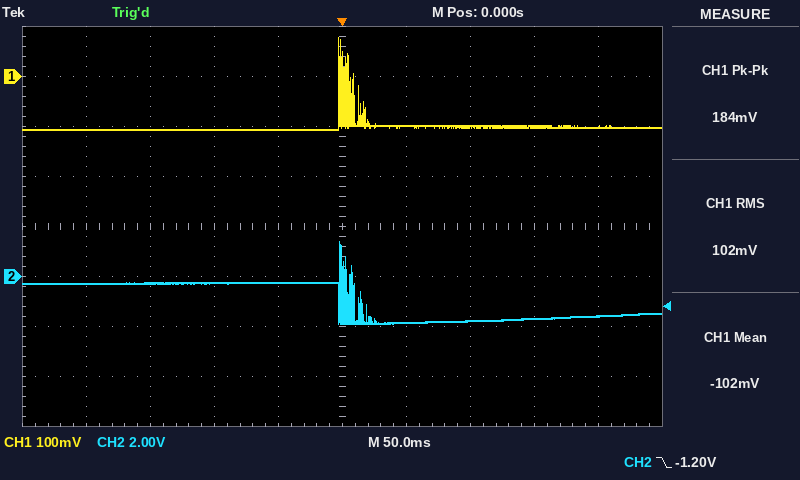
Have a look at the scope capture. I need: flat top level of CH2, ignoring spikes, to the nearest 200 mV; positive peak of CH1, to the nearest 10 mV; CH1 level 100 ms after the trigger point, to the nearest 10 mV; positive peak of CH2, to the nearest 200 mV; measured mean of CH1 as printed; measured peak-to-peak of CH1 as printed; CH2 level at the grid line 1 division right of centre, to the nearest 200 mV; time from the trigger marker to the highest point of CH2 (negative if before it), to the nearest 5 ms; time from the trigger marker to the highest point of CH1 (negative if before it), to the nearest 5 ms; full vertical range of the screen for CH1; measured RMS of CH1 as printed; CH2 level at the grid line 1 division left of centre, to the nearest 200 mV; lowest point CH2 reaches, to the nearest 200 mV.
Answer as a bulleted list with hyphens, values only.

- -200 mV
- 80 mV
- -100 mV
- 1.4 V
- -102 mV
- 184 mV
- -1.8 V
- 0 ms
- 0 ms
- 800 mV
- 102 mV
- -200 mV
- -1.8 V
